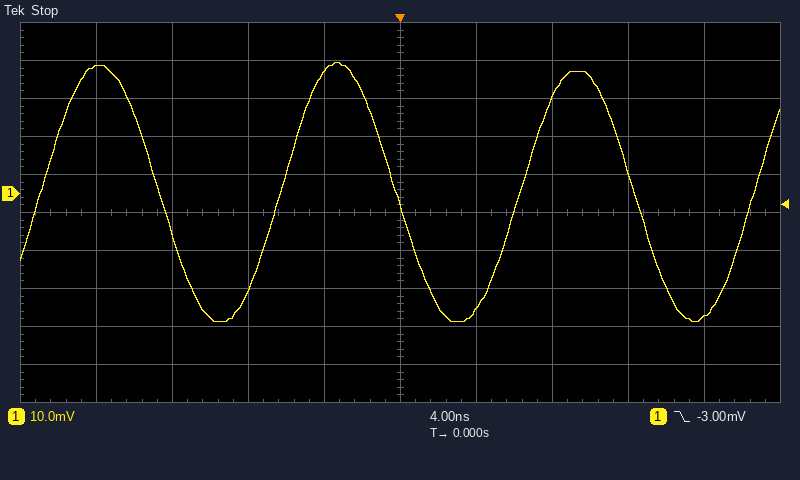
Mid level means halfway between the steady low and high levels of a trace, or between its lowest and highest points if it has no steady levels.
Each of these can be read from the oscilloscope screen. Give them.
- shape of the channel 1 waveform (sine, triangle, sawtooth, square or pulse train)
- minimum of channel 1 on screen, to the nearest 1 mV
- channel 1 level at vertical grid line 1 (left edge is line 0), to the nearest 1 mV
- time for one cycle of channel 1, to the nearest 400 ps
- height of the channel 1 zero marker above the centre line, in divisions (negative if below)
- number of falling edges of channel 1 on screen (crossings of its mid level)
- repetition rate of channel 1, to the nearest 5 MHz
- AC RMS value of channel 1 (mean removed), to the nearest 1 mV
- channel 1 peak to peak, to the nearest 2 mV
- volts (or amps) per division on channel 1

sine
-34 mV
33 mV
12.4 ns
+0.5 div
3
80 MHz
24 mV
68 mV
10 mV
